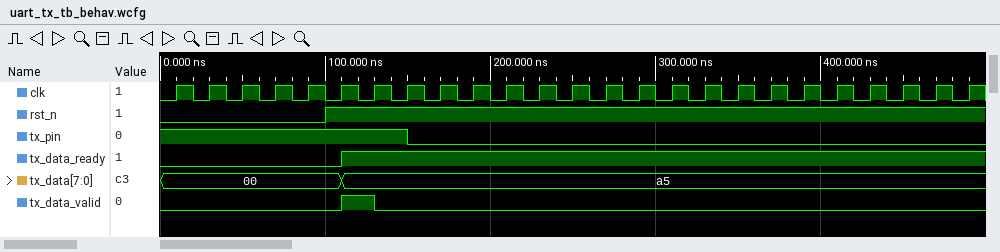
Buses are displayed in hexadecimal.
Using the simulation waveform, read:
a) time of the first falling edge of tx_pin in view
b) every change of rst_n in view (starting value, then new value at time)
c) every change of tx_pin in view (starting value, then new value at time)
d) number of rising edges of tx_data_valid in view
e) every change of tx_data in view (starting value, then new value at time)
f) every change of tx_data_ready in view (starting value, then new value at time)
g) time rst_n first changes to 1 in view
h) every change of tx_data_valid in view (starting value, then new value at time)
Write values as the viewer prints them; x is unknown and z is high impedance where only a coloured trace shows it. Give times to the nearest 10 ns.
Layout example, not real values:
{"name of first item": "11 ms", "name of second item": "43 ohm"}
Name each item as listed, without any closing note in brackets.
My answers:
{"time of the first falling edge of tx_pin in view": "150 ns", "every change of rst_n in view": "0, 1 at 100 ns", "every change of tx_pin in view": "1, 0 at 150 ns", "number of rising edges of tx_data_valid in view": "1", "every change of tx_data in view": "00, a5 at 110 ns", "every change of tx_data_ready in view": "0, 1 at 110 ns", "time rst_n first changes to 1 in view": "100 ns", "every change of tx_data_valid in view": "0, 1 at 110 ns, 0 at 130 ns"}
